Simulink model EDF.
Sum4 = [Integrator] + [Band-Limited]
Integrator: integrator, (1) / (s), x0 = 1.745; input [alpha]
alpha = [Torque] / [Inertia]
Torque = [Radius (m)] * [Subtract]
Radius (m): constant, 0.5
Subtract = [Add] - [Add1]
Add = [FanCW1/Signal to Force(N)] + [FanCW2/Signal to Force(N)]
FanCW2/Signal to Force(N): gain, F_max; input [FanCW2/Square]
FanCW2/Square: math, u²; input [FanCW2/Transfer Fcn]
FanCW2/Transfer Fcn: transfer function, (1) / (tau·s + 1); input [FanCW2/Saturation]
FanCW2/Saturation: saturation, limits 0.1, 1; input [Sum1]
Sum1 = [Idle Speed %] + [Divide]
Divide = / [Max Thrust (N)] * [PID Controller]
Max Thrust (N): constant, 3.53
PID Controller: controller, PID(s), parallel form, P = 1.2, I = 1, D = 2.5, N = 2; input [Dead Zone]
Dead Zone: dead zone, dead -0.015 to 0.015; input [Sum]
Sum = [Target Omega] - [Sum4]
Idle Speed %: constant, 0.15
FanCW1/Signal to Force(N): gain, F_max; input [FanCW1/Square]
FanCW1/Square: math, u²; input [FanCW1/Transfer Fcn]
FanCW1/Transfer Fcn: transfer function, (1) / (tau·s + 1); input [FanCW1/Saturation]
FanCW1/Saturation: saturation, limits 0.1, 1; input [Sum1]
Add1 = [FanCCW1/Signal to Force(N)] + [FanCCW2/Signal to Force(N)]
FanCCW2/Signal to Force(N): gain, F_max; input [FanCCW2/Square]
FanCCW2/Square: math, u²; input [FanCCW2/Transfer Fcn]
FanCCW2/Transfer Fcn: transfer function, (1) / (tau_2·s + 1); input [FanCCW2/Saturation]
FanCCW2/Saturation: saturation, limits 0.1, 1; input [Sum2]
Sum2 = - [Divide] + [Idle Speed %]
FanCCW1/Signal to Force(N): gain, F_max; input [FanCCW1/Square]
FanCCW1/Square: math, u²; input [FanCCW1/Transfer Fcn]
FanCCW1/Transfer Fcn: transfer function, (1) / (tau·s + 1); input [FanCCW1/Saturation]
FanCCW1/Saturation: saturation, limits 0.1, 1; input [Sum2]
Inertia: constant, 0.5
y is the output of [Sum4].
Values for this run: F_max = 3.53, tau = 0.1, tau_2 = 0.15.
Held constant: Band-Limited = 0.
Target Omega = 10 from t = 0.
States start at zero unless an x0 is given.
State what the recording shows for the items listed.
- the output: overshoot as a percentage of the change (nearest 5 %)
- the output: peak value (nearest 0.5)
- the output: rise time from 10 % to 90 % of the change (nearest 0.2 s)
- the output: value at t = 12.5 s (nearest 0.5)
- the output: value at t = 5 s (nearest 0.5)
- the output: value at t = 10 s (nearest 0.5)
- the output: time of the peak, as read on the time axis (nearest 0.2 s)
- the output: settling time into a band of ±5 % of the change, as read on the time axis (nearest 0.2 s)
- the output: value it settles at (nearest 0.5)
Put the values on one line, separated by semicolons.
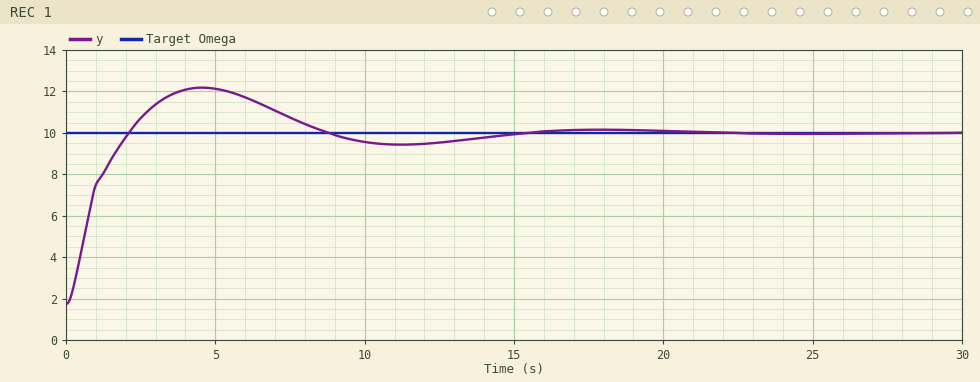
25 %; 12.0; 1.4 s; 9.5; 12.0; 9.5; 4.6 s; 12.8 s; 10.0
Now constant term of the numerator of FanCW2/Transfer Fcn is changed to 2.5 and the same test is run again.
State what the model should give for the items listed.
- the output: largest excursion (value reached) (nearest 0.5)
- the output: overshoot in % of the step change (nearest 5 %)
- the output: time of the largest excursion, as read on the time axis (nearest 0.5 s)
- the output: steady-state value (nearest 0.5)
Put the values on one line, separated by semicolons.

11.0; 15 %; 4.0 s; 10.0
